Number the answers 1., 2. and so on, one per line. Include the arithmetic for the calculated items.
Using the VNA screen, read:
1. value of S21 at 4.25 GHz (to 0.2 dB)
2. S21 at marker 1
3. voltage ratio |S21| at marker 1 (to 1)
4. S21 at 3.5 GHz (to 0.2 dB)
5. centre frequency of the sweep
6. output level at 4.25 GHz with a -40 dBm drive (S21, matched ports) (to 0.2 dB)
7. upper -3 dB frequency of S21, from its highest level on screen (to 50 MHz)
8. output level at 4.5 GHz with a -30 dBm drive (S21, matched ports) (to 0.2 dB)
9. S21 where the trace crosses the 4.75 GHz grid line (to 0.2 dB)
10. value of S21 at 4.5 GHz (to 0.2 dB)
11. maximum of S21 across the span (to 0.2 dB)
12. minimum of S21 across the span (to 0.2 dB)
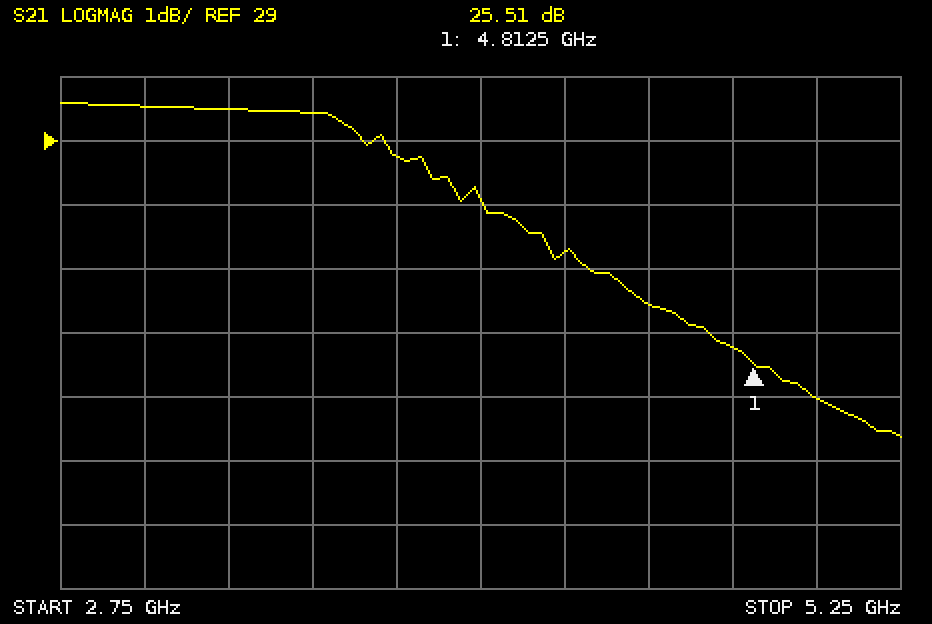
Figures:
1. 27.2 dB
2. 25.51 dB
3. 10^(25.51/20) ≈ 19
4. 29.4 dB
5. 4 GHz
6. -40 dBm + (27.2 dB) = -12.8 dBm
7. 4.45 GHz
8. -30 dBm + (26.4 dB) = -3.6 dBm
9. 25.8 dB
10. 26.4 dB
11. 29.6 dB
12. 24.4 dB
